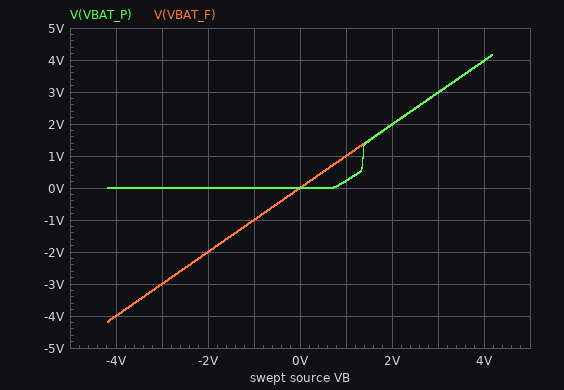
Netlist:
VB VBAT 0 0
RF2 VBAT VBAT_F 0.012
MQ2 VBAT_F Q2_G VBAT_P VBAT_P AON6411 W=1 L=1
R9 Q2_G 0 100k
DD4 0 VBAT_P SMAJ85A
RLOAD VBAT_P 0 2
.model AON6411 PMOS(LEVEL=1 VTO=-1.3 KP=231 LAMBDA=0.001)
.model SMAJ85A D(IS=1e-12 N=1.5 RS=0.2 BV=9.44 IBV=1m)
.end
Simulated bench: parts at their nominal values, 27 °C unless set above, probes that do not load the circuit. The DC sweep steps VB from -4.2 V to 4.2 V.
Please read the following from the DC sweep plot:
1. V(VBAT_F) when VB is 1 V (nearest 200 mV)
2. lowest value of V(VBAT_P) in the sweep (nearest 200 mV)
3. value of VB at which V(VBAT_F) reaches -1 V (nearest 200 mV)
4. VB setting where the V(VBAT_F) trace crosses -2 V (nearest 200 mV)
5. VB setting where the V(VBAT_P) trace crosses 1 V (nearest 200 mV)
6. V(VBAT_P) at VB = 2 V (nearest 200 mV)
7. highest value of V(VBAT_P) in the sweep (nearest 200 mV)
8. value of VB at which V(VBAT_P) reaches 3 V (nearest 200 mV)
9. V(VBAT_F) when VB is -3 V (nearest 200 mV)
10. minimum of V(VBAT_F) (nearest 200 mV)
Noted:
1.0 V
0 V
-1.0 V
-2.0 V
1.4 V
2.0 V
4.2 V
3.0 V
-3.0 V
-4.2 V
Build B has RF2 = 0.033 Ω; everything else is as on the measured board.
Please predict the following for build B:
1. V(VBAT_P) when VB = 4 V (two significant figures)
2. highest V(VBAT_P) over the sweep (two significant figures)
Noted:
3.9 V
4.1 V
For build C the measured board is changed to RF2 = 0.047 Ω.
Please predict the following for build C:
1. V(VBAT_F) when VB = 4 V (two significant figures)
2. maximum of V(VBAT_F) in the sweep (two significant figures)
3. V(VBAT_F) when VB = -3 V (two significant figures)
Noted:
3.9 V
4.1 V
-3.0 V
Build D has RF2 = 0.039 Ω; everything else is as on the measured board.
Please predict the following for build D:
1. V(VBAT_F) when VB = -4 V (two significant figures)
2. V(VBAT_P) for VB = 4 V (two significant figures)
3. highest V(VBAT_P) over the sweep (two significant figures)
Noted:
-4.0 V
3.9 V
4.1 V
